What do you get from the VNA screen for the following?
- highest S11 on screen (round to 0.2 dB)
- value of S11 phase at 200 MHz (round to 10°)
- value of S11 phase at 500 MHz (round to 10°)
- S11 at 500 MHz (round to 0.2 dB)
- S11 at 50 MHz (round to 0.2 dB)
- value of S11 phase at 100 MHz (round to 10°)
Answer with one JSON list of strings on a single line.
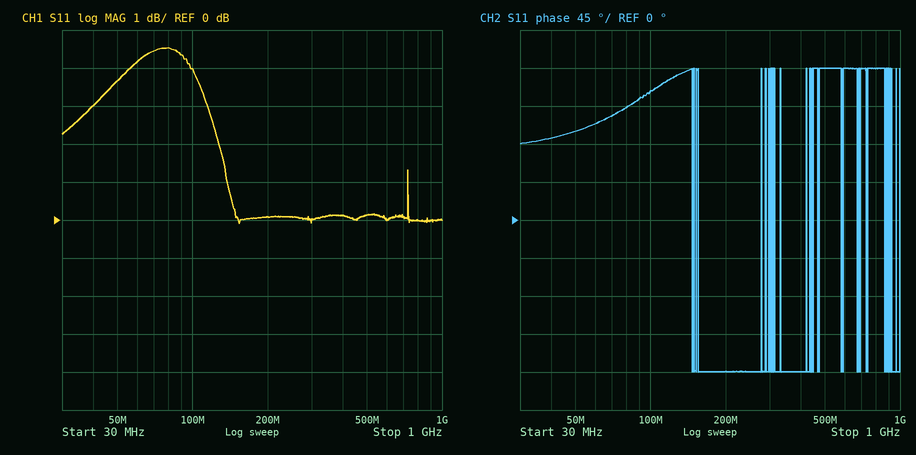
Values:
["4.6 dB", "-180°", "180°", "0.2 dB", "3.6 dB", "150°"]
